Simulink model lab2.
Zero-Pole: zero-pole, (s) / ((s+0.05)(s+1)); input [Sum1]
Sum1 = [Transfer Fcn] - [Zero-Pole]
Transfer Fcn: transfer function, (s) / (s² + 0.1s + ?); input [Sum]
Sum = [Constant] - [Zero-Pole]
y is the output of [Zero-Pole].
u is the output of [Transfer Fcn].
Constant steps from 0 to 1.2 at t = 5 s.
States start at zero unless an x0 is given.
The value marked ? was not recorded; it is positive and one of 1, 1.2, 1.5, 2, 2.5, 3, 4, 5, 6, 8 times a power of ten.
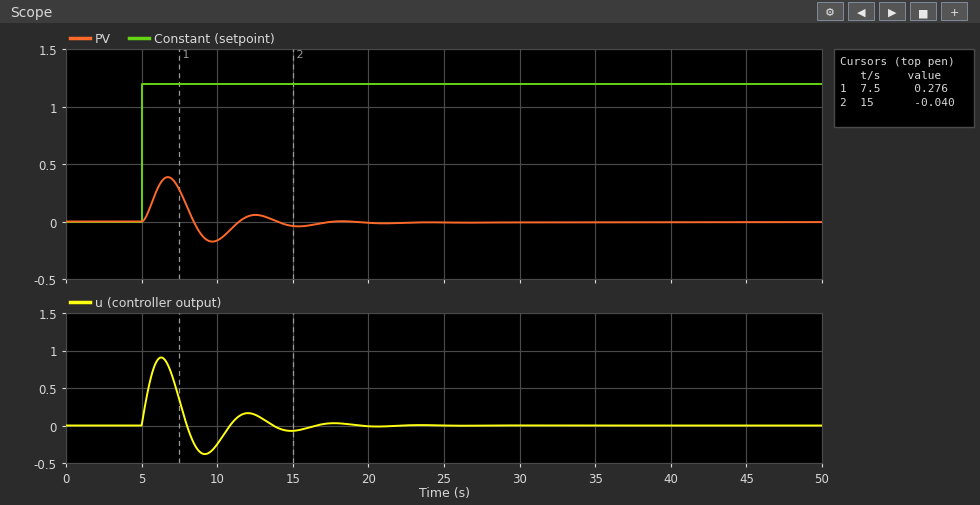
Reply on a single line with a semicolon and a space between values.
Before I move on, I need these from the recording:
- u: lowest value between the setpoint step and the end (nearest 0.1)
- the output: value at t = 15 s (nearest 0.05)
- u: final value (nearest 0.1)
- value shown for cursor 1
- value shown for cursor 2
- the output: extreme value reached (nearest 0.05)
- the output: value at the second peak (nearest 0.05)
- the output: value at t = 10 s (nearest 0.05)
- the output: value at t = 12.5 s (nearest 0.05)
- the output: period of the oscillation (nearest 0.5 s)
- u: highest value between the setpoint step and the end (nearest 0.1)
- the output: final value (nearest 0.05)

-0.4; -0.05; 0.0; 0.276; -0.040; 0.40; 0.05; -0.15; 0.05; 6.0 s; 0.9; 0.00
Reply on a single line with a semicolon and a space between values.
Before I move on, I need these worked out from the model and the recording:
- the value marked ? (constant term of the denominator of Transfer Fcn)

1
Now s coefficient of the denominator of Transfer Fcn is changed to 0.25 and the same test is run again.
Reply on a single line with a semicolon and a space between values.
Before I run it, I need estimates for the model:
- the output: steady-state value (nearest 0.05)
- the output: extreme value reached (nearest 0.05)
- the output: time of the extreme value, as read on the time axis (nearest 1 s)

0.00; 0.35; 7 s
